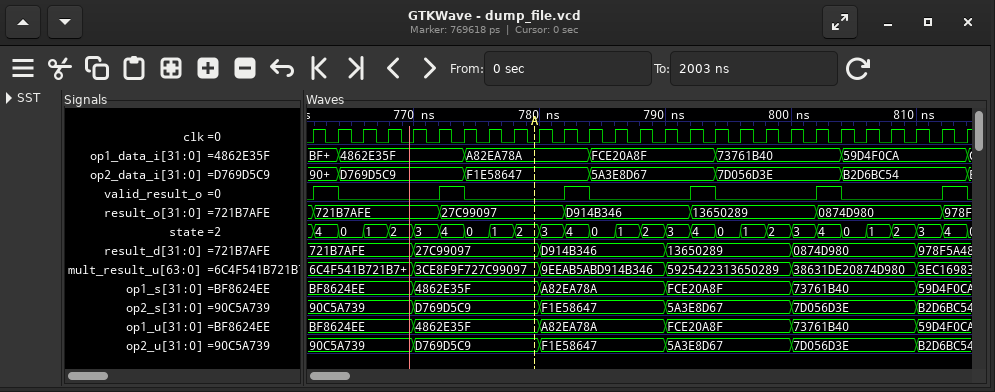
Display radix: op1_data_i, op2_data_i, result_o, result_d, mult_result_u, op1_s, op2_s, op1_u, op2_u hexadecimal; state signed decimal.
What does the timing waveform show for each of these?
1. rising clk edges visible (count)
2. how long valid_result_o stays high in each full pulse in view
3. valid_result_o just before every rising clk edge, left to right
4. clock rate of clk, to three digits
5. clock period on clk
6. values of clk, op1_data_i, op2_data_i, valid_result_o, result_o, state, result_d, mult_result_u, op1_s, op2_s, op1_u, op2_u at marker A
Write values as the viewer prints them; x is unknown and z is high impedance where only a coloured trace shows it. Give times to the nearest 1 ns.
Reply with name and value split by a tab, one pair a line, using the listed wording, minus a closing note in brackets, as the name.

rising clk edges visible	27
how long valid_result_o stays high in each full pulse in view	2 ns, 2 ns, 2 ns, 2 ns, 2 ns, 2 ns
valid_result_o just before every rising clk edge, left to right	0 1 0 0 0 0 1 0 0 0 0 1 0 0 0 0 1 0 0 0 0 1 0 0 0 0 1
clock rate of clk, to three digits	500 MHz
clock period on clk	2 ns
values of clk, op1_data_i, op2_data_i, valid_result_o, result_o, state, result_d, mult_result_u, op1_s, op2_s, op1_u, op2_u at marker A	clk=0, op1_data_i=A82EA78A, op2_data_i=F1E58647, valid_result_o=0, result_o=27C99097, state=2, result_d=27C99097, mult_result_u=3CE8F9F727C99097, op1_s=4862E35F, op2_s=D769D5C9, op1_u=4862E35F, op2_u=D769D5C9
